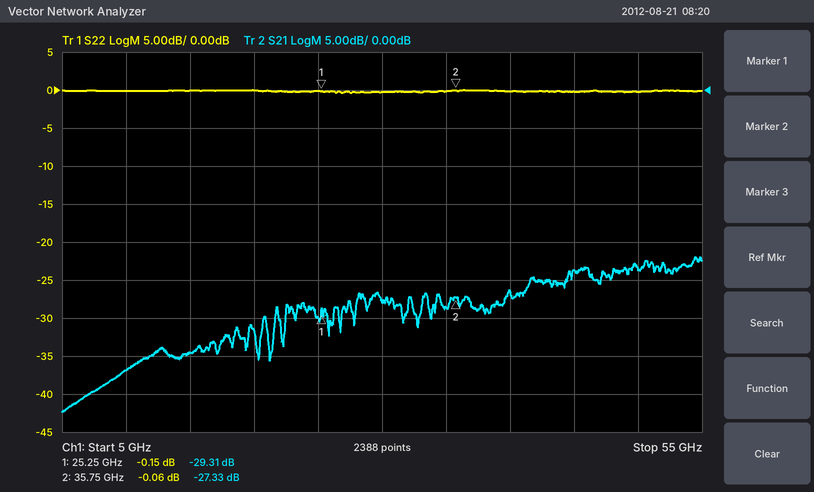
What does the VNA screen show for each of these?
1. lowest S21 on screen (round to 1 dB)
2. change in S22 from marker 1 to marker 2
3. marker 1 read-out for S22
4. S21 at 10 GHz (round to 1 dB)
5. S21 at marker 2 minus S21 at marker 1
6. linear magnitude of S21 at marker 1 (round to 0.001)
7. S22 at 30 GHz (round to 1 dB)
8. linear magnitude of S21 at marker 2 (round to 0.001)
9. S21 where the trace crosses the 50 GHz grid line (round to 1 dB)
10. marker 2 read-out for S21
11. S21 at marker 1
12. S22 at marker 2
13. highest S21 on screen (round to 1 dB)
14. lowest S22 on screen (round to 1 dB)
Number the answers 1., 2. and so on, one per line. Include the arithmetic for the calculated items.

1. -42 dB
2. -0.06 − (-0.15) = 0.09 dB
3. -0.15 dB
4. -37 dB
5. -27.33 − (-29.31) = 1.98 dB
6. 10^(-29.31/20) ≈ 0.034
7. 0 dB
8. 10^(-27.33/20) ≈ 0.043
9. -24 dB
10. -27.33 dB
11. -29.31 dB
12. -0.06 dB
13. -22 dB
14. 0 dB
